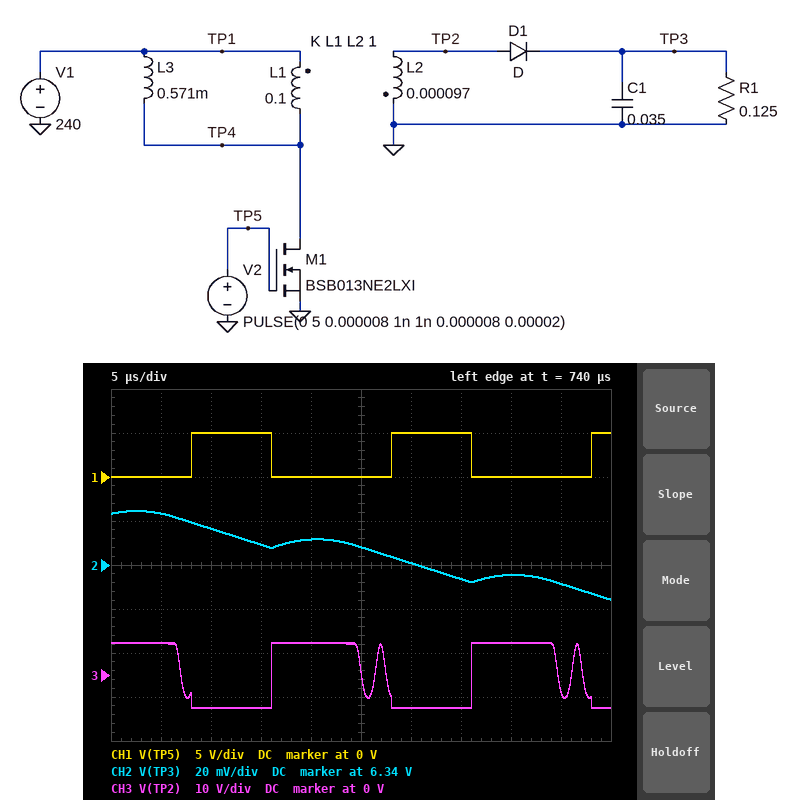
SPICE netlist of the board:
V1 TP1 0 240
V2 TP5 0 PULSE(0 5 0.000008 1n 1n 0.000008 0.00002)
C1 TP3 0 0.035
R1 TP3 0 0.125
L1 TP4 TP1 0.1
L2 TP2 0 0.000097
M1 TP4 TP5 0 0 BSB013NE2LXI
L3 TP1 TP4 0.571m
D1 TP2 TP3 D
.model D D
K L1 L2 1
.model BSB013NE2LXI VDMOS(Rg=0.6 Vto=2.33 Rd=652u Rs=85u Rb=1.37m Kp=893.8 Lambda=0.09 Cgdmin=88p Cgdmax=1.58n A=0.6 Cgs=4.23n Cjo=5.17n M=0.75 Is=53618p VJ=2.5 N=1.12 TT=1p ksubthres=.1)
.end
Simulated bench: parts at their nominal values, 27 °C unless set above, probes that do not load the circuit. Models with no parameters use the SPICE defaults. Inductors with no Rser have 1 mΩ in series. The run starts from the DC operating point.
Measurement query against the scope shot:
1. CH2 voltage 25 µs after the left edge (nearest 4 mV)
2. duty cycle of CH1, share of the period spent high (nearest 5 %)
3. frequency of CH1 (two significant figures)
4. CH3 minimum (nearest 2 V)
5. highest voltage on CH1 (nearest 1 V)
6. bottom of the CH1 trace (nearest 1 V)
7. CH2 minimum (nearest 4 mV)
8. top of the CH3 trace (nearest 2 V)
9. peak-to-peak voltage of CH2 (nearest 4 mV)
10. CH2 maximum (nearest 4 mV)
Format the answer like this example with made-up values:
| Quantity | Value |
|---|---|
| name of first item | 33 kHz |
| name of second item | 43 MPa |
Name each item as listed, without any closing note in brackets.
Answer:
| Quantity | Value |
|---|---|
| CH2 voltage 25 µs after the left edge | 6.348 V |
| duty cycle of CH1, share of the period spent high | 40 % |
| frequency of CH1 | 50 kHz |
| CH3 minimum | -8 V |
| highest voltage on CH1 | 5 V |
| bottom of the CH1 trace | 0 V |
| CH2 minimum | 6.324 V |
| top of the CH3 trace | 8 V |
| peak-to-peak voltage of CH2 | 40 mV |
| CH2 maximum | 6.364 V |
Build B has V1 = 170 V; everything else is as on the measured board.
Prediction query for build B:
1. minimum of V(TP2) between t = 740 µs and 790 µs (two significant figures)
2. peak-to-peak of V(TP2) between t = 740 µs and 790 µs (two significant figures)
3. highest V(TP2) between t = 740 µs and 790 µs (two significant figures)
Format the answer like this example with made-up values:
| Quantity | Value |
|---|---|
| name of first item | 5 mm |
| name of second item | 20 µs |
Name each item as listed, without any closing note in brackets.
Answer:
| Quantity | Value |
|---|---|
| minimum of V(TP2) between t = 740 µs and 790 µs | -5.3 V |
| peak-to-peak of V(TP2) between t = 740 µs and 790 µs | 10 V |
| highest V(TP2) between t = 740 µs and 790 µs | 5.0 V |
